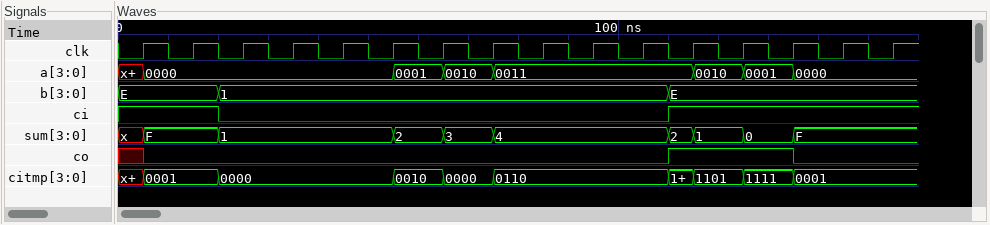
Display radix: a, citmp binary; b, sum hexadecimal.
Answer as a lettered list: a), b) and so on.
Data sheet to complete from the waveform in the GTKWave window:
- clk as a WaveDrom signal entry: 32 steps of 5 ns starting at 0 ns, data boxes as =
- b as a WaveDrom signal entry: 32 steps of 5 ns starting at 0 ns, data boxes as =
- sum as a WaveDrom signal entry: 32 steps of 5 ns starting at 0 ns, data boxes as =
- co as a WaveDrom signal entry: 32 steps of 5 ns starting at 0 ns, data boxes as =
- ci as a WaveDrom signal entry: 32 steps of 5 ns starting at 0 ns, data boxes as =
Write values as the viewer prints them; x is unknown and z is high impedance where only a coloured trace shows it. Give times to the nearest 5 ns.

a) {name: 'clk', wave: '01010101010101010101010101010101'}
b) {name: 'b', wave: '=...=.................=.........', data: 'E 1 E'}
c) {name: 'sum', wave: 'x=..=......=.=.=......==.=.=....', data: 'F 1 2 3 4 2 1 0 F'}
d) {name: 'co', wave: 'x0....................1....0....'}
e) {name: 'ci', wave: '1...0.................1.........'}
